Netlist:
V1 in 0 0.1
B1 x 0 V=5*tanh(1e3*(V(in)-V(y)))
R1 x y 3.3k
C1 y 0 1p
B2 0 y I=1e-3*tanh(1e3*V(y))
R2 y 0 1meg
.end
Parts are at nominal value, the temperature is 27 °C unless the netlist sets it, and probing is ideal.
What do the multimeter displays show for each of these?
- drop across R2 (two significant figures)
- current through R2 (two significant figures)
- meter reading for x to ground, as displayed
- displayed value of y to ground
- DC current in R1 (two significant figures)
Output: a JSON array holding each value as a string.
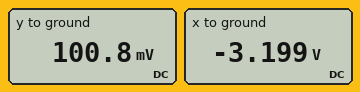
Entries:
["100 mV", "100 nA", "-3.199 V", "100.8 mV", "1.0 mA"]
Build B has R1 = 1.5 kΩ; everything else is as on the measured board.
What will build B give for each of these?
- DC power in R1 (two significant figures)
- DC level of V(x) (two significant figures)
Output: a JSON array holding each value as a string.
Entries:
["1.5 mW", "-1.4 V"]
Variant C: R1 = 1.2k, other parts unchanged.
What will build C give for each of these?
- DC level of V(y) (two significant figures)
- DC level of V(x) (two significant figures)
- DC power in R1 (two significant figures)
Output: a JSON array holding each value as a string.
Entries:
["100 mV", "-1.1 V", "1.2 mW"]
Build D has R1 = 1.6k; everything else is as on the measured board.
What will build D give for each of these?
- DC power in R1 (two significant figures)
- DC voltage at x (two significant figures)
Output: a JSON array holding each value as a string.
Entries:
["1.6 mW", "-1.5 V"]
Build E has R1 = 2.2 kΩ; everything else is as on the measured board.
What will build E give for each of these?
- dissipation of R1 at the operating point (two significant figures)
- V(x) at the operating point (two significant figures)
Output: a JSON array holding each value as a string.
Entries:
["2.2 mW", "-2.1 V"]
